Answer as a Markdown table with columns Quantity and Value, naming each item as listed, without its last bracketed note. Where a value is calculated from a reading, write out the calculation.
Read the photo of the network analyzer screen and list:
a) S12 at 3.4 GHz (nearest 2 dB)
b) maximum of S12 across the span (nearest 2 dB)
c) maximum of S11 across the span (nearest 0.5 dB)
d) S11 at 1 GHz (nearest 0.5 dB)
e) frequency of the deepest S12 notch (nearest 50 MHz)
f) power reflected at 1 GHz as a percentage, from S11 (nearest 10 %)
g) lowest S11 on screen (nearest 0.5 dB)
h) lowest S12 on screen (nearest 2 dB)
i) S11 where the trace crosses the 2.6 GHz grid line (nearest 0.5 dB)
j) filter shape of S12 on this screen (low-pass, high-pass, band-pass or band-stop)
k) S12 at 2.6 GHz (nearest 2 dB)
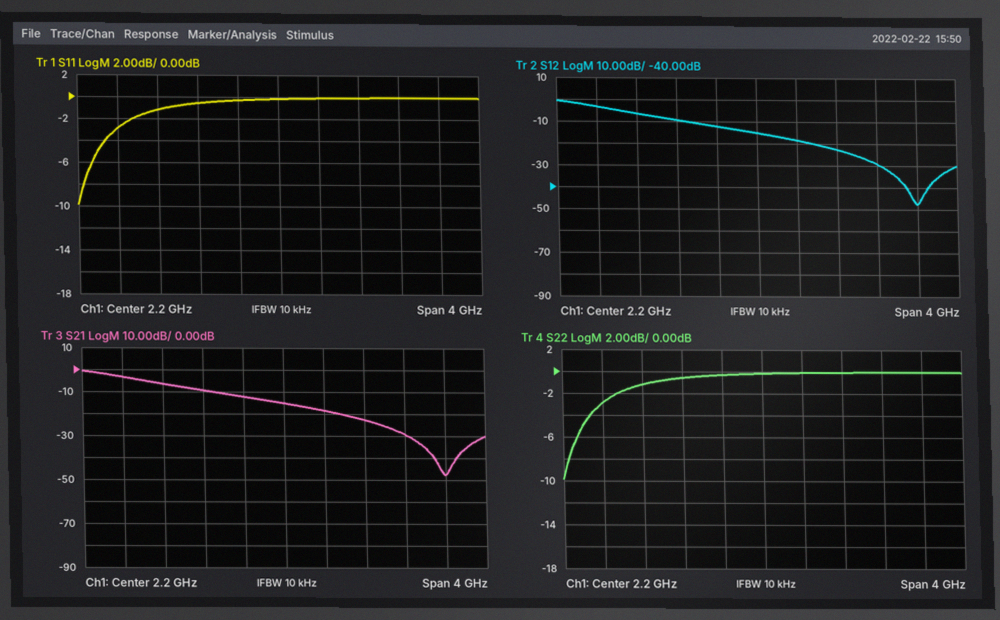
| Quantity | Value |
|---|---|
| S12 at 3.4 GHz | -30 dB |
| maximum of S12 across the span | 0 dB |
| maximum of S11 across the span | 0.0 dB |
| S11 at 1 GHz | -1.0 dB |
| frequency of the deepest S12 notch | 3.80 GHz |
| power reflected at 1 GHz as a percentage, from S11 | 10^(-1/10) ≈ 79.4 %, so 80 % to the nearest 10 % |
| lowest S11 on screen | -10.0 dB |
| lowest S12 on screen | -48 dB |
| S11 where the trace crosses the 2.6 GHz grid line | 0.0 dB |
| filter shape of S12 on this screen | low-pass |
| S12 at 2.6 GHz | -18 dB |
